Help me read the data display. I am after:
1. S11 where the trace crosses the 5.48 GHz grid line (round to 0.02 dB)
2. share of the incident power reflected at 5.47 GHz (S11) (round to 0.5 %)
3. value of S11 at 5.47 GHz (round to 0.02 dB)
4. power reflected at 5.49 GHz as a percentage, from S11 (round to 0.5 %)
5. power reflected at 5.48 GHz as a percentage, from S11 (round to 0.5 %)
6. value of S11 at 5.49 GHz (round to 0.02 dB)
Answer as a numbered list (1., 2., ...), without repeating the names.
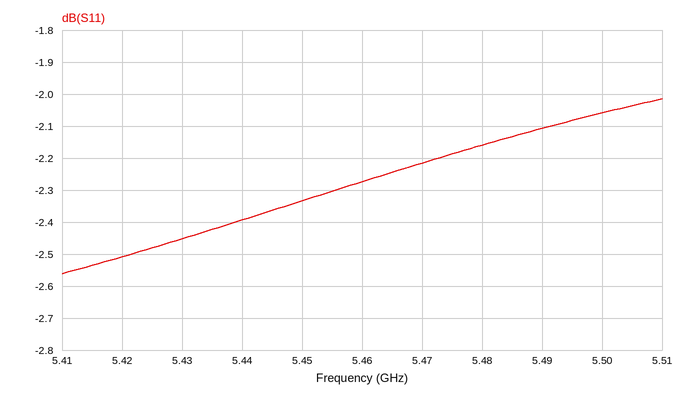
1. -2.16 dB
2. 60.0 %
3. -2.22 dB
4. 61.5 %
5. 61.0 %
6. -2.10 dB
